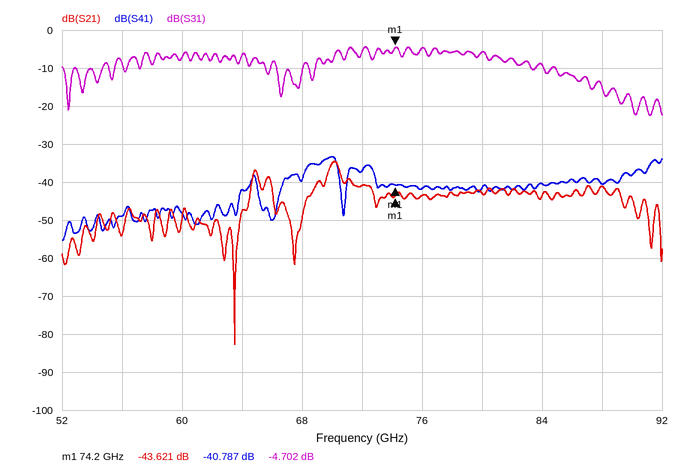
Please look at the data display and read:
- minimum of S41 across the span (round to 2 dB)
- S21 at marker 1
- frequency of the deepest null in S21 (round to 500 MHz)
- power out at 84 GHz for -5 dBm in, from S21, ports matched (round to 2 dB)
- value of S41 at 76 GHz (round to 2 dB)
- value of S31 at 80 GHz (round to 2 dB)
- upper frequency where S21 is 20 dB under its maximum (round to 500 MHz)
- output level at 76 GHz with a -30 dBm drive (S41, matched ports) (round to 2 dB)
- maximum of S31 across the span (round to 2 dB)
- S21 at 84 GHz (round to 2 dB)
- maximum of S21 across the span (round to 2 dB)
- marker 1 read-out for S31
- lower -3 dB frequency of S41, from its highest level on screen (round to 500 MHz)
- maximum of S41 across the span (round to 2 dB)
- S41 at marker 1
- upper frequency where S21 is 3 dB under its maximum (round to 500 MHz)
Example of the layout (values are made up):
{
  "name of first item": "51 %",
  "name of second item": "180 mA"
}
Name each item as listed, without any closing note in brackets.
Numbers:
{
  "minimum of S41 across the span": "-56 dB",
  "S21 at marker 1": "-43.621 dB",
  "frequency of the deepest null in S21": "63.5 GHz",
  "power out at 84 GHz for -5 dBm in, from S21, ports matched": "-48 dBm",
  "value of S41 at 76 GHz": "-42 dB",
  "value of S31 at 80 GHz": "-6 dB",
  "upper frequency where S21 is 20 dB under its maximum": "91.0 GHz",
  "output level at 76 GHz with a -30 dBm drive (S41, matched ports)": "-72 dBm",
  "maximum of S31 across the span": "-4 dB",
  "S21 at 84 GHz": "-44 dB",
  "maximum of S21 across the span": "-34 dB",
  "marker 1 read-out for S31": "-4.702 dB",
  "lower -3 dB frequency of S41, from its highest level on screen": "68.5 GHz",
  "maximum of S41 across the span": "-34 dB",
  "S41 at marker 1": "-40.787 dB",
  "upper frequency where S21 is 3 dB under its maximum": "70.5 GHz"
}
